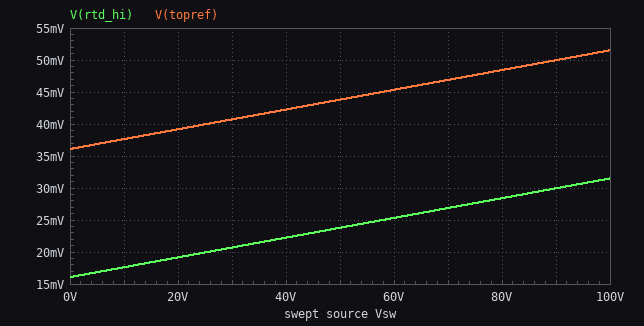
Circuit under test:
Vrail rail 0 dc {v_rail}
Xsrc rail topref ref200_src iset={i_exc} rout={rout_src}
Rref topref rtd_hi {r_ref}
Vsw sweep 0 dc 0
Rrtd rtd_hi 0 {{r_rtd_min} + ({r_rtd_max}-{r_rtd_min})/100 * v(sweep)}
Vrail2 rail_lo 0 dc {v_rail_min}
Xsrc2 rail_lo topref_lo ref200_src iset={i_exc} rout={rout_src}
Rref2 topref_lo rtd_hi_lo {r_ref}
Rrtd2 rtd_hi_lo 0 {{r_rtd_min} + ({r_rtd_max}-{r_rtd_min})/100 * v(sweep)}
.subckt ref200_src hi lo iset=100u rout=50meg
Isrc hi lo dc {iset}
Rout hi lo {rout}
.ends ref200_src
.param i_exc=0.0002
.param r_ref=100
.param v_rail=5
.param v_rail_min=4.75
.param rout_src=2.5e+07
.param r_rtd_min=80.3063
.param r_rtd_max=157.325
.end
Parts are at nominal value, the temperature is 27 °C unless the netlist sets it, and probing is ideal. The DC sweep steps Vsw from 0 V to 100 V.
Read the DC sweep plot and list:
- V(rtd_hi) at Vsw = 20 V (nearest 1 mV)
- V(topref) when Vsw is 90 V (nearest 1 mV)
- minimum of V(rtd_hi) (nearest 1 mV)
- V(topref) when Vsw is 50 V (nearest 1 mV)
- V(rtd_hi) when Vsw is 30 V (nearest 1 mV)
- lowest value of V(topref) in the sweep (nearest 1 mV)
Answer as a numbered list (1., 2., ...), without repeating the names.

1. 19 mV
2. 50 mV
3. 16 mV
4. 44 mV
5. 21 mV
6. 36 mV
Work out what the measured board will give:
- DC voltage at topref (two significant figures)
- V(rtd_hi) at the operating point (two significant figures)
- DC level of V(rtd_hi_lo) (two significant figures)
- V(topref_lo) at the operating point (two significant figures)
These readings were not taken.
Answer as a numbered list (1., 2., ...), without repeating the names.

1. 36 mV
2. 16 mV
3. 16 mV
4. 36 mV
